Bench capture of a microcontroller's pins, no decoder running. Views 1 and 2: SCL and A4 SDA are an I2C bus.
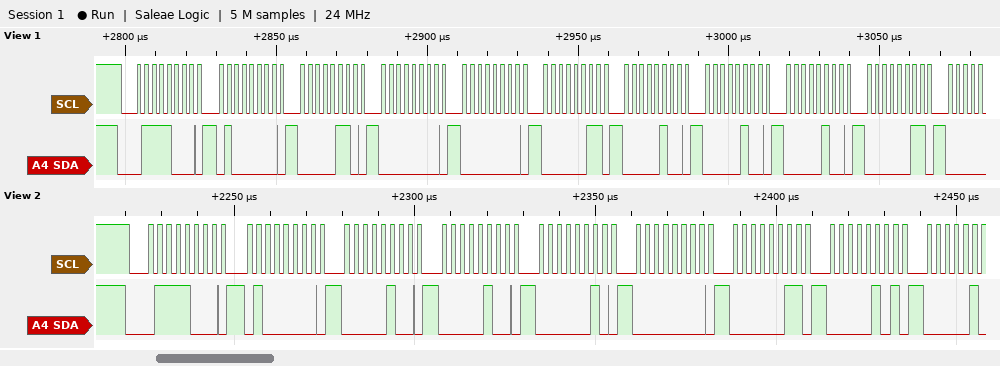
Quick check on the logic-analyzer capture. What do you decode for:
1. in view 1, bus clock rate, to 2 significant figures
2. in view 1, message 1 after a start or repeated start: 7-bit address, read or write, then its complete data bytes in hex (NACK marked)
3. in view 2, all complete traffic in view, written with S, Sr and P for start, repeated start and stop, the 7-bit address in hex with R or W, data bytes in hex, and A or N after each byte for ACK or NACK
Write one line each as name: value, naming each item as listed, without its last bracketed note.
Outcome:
in view 1, bus clock rate, to 2 significant figures: 400 kHz
in view 1, message 1 after a start or repeated start: 7-bit address, read or write, then its complete data bytes in hex: 0x3C write: 40 06 00 00 03 04 04 04 03
in view 2, all complete traffic in view, written with S, Sr and P for start, repeated start and stop, the 7-bit address in hex with R or W, data bytes in hex, and A or N after each byte for ACK or NACK: S 3CW A 40 A 04 A 04 A 02 A 00 A 03 A 05 A
